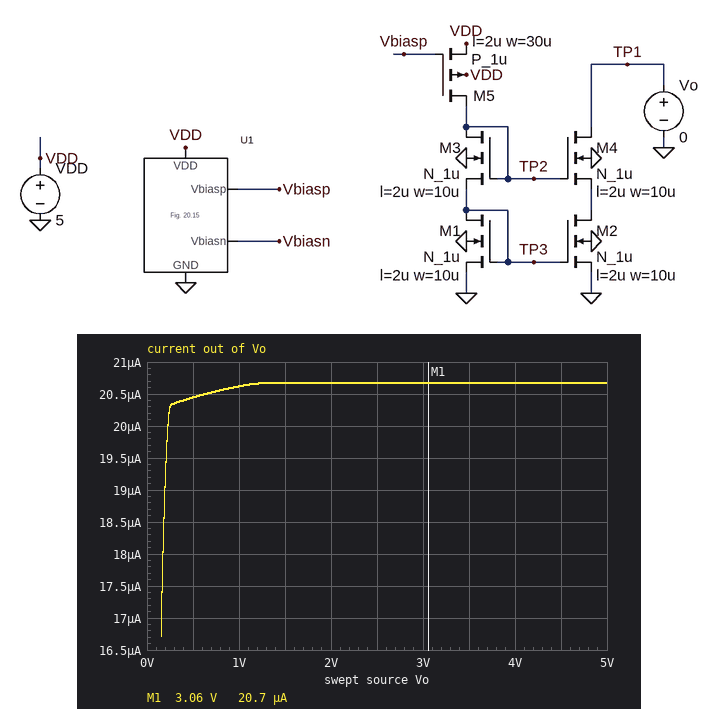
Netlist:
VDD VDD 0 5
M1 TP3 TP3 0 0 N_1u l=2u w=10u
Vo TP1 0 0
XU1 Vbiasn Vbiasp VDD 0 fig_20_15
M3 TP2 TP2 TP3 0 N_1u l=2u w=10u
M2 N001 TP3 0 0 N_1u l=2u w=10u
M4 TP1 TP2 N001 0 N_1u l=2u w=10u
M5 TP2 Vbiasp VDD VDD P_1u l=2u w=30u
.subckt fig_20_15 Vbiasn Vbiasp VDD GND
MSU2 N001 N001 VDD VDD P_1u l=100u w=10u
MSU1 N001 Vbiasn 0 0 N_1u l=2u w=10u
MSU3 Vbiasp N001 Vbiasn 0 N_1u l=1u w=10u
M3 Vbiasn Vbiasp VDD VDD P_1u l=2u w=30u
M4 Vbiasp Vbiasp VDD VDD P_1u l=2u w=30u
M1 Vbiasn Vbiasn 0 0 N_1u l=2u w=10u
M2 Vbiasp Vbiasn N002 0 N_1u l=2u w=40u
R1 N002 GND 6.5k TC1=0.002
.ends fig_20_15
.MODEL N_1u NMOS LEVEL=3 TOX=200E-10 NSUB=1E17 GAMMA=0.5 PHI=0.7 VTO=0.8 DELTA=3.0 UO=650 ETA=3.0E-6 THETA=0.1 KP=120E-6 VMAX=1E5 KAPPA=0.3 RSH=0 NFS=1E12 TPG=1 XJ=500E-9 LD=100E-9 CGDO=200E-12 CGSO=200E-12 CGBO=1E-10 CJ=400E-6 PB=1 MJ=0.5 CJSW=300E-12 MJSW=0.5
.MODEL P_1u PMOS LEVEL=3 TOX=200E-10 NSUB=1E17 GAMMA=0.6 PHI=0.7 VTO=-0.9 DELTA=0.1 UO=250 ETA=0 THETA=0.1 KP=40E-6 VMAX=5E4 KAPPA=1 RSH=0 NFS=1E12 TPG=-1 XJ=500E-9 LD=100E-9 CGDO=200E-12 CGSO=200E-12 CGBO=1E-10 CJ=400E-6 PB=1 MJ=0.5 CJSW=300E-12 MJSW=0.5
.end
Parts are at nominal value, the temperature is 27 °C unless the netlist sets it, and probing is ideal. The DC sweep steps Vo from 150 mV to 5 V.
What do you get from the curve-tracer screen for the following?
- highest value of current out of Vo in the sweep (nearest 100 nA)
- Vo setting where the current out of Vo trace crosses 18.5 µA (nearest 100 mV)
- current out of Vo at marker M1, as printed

20.7 µA
200 mV
20.7 µA
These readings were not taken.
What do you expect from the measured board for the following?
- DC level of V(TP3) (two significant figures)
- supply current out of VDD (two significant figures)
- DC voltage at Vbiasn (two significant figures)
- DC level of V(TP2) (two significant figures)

1.1 V
81 µA
1.1 V
2.4 V
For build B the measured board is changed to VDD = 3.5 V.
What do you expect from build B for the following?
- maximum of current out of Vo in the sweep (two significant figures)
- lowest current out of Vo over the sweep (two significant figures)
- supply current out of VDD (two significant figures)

19 µA
16 µA
67 µA
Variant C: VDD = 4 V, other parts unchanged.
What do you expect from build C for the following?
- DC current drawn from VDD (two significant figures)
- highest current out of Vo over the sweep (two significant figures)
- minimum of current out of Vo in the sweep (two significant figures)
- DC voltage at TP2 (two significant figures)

71 µA
20 µA
16 µA
2.4 V
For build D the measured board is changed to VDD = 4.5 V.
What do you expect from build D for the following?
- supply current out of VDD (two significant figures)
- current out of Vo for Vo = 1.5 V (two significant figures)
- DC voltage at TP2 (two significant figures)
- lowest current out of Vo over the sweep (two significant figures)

76 µA
20 µA
2.4 V
16 µA
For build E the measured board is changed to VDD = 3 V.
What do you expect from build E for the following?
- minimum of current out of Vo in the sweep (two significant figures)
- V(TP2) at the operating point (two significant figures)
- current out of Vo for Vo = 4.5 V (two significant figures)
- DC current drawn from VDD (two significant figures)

16 µA
2.4 V
19 µA
63 µA
